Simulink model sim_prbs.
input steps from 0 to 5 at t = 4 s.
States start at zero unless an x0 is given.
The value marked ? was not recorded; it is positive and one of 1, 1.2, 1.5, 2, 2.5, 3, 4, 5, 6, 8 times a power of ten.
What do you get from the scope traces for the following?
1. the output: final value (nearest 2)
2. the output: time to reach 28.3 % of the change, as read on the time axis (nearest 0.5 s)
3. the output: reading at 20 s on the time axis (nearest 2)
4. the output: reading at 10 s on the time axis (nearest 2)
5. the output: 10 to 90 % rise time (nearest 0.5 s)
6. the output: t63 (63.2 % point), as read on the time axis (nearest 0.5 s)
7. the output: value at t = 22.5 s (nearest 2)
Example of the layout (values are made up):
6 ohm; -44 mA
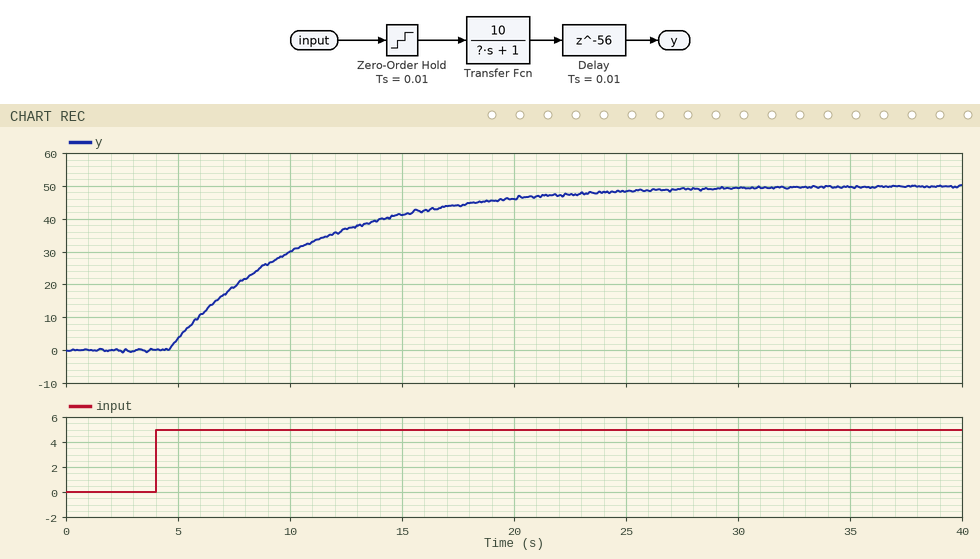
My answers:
50; 6.5 s; 46; 30; 13.0 s; 10.5 s; 48
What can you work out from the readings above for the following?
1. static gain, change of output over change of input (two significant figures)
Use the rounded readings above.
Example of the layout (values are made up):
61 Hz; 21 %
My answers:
10
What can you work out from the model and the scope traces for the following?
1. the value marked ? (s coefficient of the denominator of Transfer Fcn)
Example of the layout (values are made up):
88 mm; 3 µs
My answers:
6
